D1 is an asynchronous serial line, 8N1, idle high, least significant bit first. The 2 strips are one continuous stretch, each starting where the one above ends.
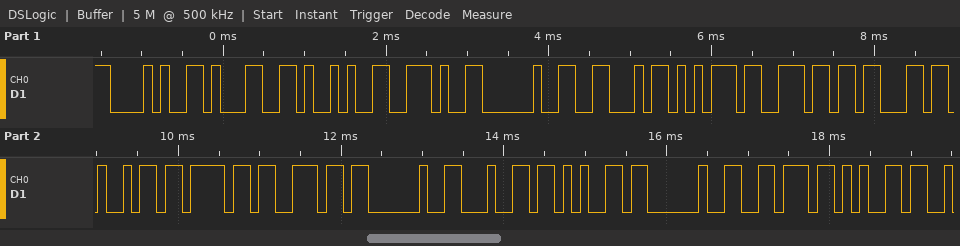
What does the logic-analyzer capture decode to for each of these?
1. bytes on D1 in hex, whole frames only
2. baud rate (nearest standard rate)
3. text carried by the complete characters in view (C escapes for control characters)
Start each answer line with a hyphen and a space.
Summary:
- 28 31 29 2E 20 46 75 6E 63 69 6F 6E 20 64 65 20 76 65
- 9600 baud
- "(1). Funcion de ve"
